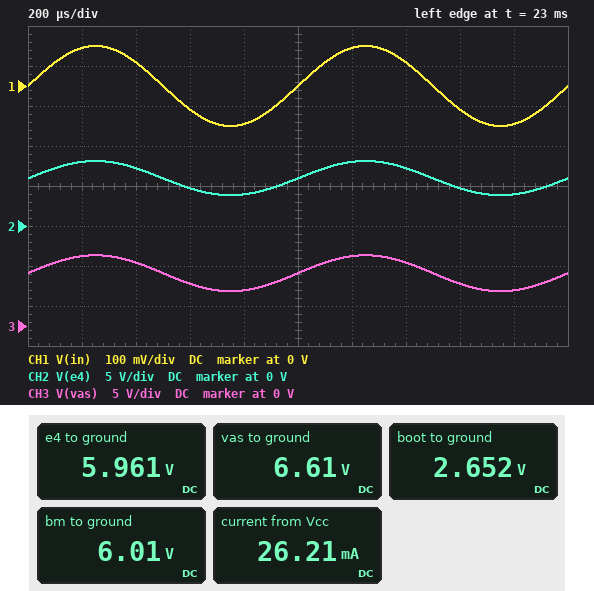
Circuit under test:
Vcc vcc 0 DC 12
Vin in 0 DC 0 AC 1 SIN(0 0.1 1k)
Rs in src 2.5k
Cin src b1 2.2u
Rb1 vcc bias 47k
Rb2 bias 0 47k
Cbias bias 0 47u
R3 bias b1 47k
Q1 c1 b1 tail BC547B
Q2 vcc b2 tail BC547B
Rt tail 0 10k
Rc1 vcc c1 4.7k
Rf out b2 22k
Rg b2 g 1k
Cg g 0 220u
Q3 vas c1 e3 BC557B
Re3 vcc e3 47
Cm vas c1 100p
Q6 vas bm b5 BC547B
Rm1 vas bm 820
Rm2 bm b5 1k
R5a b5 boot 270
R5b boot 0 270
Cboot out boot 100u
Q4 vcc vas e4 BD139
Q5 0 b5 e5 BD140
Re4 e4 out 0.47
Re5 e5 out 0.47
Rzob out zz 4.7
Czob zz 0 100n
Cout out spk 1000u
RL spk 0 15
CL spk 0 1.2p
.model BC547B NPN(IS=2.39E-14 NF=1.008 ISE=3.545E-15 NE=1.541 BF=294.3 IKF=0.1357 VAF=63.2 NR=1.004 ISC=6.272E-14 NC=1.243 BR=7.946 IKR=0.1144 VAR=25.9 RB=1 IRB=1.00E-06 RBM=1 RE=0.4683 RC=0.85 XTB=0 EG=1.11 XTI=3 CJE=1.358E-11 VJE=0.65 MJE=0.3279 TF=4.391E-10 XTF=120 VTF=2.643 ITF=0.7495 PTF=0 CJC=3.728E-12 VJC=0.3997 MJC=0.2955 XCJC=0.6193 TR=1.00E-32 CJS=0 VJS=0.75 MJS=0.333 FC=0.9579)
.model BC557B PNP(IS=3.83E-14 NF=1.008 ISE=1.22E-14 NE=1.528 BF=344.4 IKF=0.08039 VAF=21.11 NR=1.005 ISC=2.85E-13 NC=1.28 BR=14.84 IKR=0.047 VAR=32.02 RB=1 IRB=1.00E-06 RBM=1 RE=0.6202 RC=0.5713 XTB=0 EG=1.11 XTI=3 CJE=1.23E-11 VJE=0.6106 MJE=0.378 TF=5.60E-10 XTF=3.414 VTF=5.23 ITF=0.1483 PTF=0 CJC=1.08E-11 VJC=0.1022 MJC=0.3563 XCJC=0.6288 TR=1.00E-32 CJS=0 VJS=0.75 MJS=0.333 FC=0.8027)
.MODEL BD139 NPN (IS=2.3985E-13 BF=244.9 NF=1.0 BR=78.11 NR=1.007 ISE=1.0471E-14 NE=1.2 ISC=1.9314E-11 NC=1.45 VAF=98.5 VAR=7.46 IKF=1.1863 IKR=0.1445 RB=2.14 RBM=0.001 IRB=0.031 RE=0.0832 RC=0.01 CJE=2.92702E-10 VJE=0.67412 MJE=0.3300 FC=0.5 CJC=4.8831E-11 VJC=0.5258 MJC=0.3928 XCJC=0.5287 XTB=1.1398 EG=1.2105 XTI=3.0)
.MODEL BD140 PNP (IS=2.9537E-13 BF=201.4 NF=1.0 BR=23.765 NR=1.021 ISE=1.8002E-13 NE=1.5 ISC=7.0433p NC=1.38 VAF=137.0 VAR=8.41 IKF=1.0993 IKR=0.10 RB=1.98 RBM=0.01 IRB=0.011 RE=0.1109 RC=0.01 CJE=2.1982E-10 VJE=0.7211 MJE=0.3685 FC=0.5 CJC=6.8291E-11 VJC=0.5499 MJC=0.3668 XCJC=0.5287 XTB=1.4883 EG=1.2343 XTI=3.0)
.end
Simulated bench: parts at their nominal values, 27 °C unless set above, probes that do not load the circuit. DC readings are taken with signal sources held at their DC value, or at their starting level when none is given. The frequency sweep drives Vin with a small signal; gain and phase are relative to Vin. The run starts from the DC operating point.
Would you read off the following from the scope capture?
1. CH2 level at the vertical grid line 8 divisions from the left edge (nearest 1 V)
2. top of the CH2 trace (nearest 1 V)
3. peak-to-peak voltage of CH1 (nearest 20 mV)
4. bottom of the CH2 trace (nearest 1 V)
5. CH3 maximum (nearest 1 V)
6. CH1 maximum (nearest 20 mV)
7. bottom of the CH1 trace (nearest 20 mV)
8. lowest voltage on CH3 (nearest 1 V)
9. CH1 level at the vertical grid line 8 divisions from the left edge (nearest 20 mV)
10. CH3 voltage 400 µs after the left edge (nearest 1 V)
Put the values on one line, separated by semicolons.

5 V; 8 V; 200 mV; 4 V; 9 V; 100 mV; -100 mV; 4 V; -60 mV; 8 V
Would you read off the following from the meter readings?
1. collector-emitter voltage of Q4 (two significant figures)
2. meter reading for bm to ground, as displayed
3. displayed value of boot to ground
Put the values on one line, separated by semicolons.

6.0 V; 6.01 V; 2.652 V
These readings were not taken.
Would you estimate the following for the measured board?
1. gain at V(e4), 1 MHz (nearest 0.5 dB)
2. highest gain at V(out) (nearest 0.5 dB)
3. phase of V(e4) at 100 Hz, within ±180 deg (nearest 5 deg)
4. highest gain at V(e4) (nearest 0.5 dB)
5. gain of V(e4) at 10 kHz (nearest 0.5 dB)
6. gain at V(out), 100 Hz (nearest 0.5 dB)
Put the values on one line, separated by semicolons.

14.0 dB; 26.5 dB; 0 deg; 26.5 dB; 26.5 dB; 26.5 dB
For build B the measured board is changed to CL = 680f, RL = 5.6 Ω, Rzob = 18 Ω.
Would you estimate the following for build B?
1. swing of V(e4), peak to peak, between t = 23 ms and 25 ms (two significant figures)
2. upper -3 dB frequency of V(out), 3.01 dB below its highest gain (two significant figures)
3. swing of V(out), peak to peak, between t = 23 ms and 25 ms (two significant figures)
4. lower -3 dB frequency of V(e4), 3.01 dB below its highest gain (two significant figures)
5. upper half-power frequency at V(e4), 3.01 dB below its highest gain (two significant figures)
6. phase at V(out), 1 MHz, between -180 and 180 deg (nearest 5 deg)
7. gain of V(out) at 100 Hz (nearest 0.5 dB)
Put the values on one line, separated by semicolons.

4.1 V; 250 kHz; 3.9 V; 2.1 Hz; 270 kHz; -105 deg; 26.0 dB
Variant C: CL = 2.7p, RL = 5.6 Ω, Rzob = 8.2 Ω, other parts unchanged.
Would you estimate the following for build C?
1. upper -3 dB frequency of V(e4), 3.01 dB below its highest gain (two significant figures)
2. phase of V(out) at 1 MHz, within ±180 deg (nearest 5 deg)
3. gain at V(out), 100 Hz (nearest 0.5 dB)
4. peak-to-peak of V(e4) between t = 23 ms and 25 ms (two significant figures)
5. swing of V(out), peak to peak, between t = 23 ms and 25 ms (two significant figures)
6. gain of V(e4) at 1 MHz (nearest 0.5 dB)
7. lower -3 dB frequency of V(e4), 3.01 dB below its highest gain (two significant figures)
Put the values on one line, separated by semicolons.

270 kHz; -105 deg; 26.0 dB; 4.1 V; 3.9 V; 13.5 dB; 2.1 Hz
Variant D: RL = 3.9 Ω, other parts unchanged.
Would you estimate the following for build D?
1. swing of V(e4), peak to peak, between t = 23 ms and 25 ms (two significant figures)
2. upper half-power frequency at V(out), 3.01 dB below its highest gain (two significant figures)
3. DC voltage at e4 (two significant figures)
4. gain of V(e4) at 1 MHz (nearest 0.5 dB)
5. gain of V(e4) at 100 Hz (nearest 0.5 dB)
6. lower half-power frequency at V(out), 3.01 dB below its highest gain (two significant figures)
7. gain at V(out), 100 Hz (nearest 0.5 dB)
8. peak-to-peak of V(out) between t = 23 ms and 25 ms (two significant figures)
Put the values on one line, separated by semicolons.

3.9 V; 220 kHz; 6.0 V; 12.5 dB; 26.0 dB; 2.1 Hz; 25.5 dB; 3.7 V
